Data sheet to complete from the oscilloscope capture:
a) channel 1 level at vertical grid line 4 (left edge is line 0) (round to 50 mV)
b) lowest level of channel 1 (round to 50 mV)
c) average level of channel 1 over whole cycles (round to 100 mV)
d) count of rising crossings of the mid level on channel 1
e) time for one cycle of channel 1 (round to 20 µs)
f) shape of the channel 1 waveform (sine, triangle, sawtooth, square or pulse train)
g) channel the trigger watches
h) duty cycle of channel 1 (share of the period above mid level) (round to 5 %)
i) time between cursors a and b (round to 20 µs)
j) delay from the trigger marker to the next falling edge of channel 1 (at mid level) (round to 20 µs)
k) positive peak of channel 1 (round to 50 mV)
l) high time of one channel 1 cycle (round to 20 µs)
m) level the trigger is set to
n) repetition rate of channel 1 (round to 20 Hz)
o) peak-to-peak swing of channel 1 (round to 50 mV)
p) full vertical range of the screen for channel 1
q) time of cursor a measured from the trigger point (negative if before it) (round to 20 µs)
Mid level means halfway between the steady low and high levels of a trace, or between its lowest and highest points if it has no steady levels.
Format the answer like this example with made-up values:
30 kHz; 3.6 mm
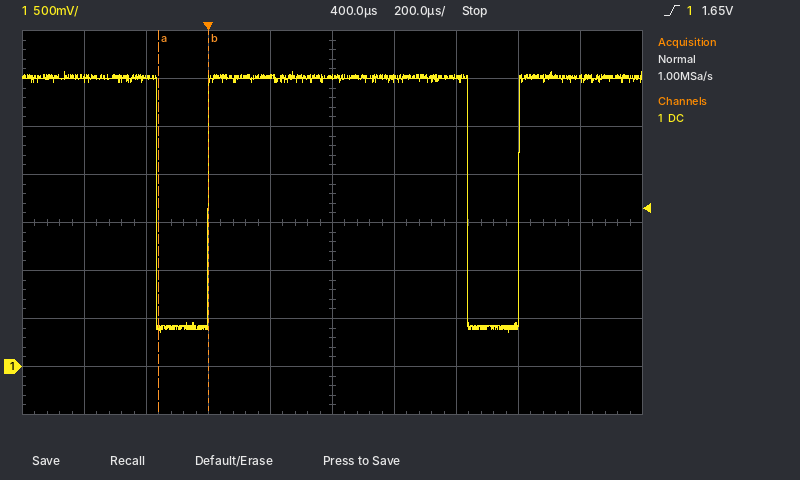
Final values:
3.00 V; 350 mV; 2.6 V; 2; 1.00 ms; pulse train; channel 1; 85 %; 160 µs; 840 µs; 3.05 V; 840 µs; 1.65 V; 1.00 kHz; 2.70 V; 4 V; -160 µs
